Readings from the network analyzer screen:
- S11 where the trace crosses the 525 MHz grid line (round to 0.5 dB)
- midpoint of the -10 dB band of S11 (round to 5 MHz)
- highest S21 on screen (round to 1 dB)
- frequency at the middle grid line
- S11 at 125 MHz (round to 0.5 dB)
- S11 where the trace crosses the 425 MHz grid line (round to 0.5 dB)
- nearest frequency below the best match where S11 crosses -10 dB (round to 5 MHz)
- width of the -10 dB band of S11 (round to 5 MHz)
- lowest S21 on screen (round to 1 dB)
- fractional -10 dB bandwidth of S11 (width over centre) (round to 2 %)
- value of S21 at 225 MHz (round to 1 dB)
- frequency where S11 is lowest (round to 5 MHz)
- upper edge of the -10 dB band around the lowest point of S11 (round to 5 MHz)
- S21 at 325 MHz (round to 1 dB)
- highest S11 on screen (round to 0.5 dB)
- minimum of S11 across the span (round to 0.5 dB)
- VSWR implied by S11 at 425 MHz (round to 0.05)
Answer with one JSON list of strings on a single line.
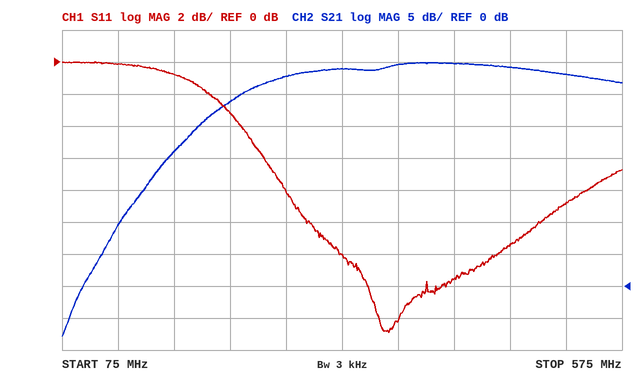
["-9.0 dB", "400 MHz", "35 dB", "325 MHz", "0.0 dB", "-13.5 dB", "295 MHz", "205 MHz", "-8 dB", "52 %", "29 dB", "365 MHz", "500 MHz", "34 dB", "0.0 dB", "-17.0 dB", "1.55"]
